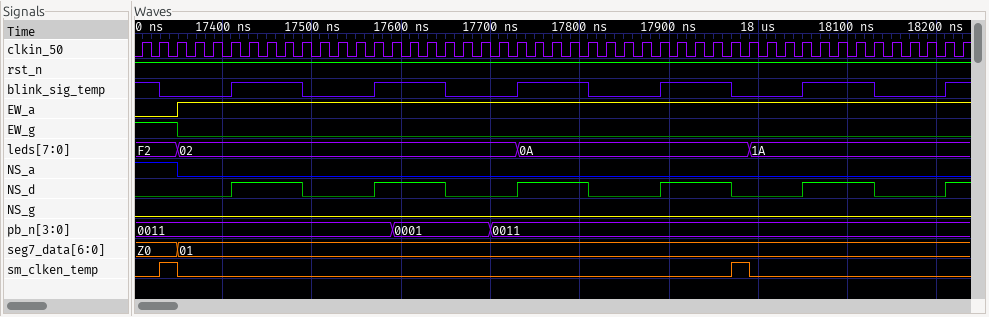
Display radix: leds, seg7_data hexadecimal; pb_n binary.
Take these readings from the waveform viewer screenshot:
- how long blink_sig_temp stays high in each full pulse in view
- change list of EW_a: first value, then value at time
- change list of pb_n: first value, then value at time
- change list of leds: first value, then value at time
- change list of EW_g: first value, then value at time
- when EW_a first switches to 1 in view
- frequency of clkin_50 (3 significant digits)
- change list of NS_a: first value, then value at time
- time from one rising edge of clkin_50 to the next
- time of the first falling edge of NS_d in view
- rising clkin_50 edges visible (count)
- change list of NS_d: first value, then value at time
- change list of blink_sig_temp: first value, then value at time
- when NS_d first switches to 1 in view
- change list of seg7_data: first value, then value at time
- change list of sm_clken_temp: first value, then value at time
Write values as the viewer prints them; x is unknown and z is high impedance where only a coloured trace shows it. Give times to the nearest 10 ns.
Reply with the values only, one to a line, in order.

80 ns, 80 ns, 80 ns, 80 ns, 80 ns
0, 1 at 17350 ns
0011, 0001 at 17590 ns, 0011 at 17700 ns
F2, 02 at 17350 ns, 0A at 17730 ns, 1A at 17990 ns
1, 0 at 17350 ns
17350 ns
50.0 MHz
1, 0 at 17350 ns
20 ns
17490 ns
47
0, 1 at 17410 ns, 0 at 17490 ns, 1 at 17570 ns, 0 at 17650 ns, 1 at 17730 ns, 0 at 17810 ns, 1 at 17890 ns, 0 at 17970 ns, 1 at 18050 ns, 0 at 18130 ns, 1 at 18210 ns
1, 0 at 17330 ns, 1 at 17410 ns, 0 at 17490 ns, 1 at 17570 ns, 0 at 17650 ns, 1 at 17730 ns, 0 at 17810 ns, 1 at 17890 ns, 0 at 17970 ns, 1 at 18050 ns, 0 at 18130 ns, 1 at 18210 ns
17410 ns
Z0, 01 at 17350 ns
0, 1 at 17330 ns, 0 at 17350 ns, 1 at 17970 ns, 0 at 17990 ns
